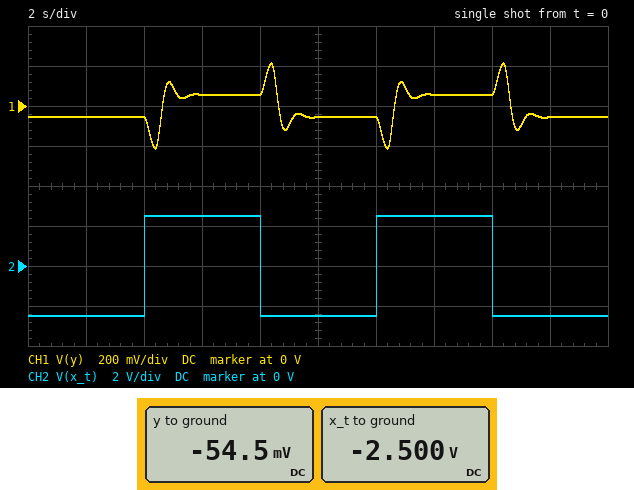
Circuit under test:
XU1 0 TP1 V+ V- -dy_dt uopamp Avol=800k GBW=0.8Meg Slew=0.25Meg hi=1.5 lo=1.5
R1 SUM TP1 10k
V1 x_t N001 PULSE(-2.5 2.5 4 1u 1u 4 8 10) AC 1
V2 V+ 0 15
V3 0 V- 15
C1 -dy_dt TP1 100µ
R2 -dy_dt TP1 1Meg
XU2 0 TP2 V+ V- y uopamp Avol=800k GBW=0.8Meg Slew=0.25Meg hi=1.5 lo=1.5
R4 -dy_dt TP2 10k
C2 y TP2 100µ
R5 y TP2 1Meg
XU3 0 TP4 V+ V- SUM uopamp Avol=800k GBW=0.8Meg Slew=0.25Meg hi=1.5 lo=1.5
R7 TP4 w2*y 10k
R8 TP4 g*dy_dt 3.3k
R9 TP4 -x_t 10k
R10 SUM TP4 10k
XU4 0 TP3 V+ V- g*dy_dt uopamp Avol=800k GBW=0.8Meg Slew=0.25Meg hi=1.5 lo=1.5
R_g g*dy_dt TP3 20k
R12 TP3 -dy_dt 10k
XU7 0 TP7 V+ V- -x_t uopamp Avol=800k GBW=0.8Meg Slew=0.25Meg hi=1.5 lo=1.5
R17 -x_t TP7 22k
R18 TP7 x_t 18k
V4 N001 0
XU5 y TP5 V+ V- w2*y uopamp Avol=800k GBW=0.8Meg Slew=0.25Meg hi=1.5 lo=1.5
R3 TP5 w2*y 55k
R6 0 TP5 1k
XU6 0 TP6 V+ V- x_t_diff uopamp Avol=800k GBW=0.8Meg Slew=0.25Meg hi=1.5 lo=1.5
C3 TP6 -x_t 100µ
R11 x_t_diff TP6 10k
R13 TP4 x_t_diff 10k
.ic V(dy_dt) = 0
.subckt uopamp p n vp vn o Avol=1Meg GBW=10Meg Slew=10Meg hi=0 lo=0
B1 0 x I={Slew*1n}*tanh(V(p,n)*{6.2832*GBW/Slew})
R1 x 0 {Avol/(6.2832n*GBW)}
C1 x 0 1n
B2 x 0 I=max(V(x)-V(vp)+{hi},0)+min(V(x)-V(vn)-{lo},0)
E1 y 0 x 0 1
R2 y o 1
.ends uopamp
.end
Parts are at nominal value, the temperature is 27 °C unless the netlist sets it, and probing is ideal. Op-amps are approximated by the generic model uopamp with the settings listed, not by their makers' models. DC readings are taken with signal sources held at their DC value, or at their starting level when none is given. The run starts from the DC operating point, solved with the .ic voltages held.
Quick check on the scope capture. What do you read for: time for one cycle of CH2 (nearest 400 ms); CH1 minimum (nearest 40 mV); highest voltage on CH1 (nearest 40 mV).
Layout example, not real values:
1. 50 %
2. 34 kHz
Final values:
1. 8.0 s
2. -200 mV
3. 200 mV
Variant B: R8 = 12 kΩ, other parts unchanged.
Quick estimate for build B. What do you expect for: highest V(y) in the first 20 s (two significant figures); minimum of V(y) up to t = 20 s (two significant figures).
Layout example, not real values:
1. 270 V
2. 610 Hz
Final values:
1. 290 mV
2. -290 mV
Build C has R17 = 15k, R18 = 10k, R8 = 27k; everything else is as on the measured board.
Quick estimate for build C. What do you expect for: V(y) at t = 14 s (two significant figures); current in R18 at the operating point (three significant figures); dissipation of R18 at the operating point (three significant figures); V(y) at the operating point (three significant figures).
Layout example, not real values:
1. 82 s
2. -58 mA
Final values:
1. 310 mV
2. 250 µA
3. 625 µW
4. -67.0 mV
